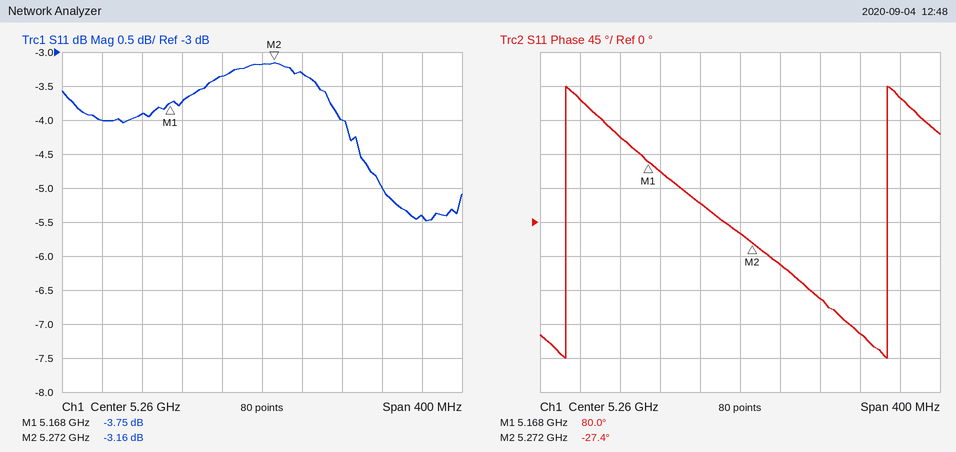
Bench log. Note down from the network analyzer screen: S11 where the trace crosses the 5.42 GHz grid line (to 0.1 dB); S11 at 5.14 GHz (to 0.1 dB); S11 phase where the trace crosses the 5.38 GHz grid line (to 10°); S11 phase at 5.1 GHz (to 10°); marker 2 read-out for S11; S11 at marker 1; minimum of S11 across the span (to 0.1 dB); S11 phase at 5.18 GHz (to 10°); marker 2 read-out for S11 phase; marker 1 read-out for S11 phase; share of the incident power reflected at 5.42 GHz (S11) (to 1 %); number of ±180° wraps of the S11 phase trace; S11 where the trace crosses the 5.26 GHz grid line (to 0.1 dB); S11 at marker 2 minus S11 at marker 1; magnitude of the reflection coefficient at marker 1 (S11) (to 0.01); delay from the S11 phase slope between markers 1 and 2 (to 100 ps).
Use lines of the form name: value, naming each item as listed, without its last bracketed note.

S11 where the trace crosses the 5.42 GHz grid line: -5.4 dB
S11 at 5.14 GHz: -3.9 dB
S11 phase where the trace crosses the 5.38 GHz grid line: -150°
S11 phase at 5.1 GHz: 160°
marker 2 read-out for S11: -3.16 dB
S11 at marker 1: -3.75 dB
minimum of S11 across the span: -5.5 dB
S11 phase at 5.18 GHz: 70°
marker 2 read-out for S11 phase: -27.4°
marker 1 read-out for S11 phase: 80.0°
share of the incident power reflected at 5.42 GHz (S11): 29 %
number of ±180° wraps of the S11 phase trace: 2
S11 where the trace crosses the 5.26 GHz grid line: -3.2 dB
S11 at marker 2 minus S11 at marker 1: 0.59 dB
magnitude of the reflection coefficient at marker 1 (S11): 0.65
delay from the S11 phase slope between markers 1 and 2: 2.9 ns
